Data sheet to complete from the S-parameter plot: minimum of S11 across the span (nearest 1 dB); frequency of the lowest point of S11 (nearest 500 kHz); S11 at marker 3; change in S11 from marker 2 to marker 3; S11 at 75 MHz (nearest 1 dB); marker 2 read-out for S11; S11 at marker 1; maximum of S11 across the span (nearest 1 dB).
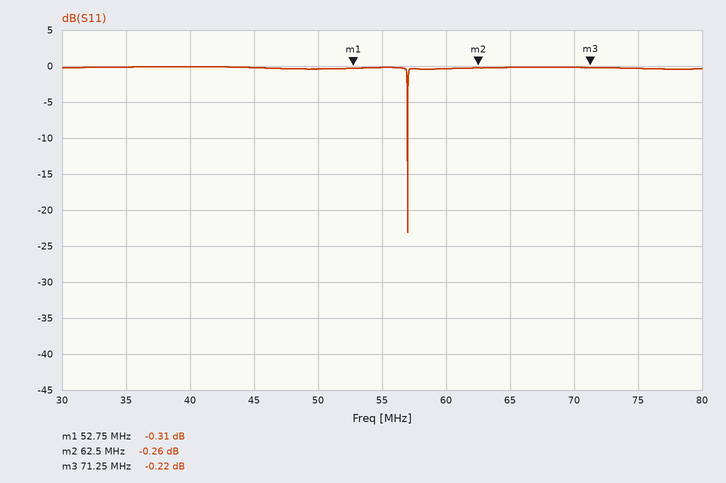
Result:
-23 dB
57.0 MHz
-0.22 dB
0.04 dB
0 dB
-0.26 dB
-0.31 dB
0 dB
